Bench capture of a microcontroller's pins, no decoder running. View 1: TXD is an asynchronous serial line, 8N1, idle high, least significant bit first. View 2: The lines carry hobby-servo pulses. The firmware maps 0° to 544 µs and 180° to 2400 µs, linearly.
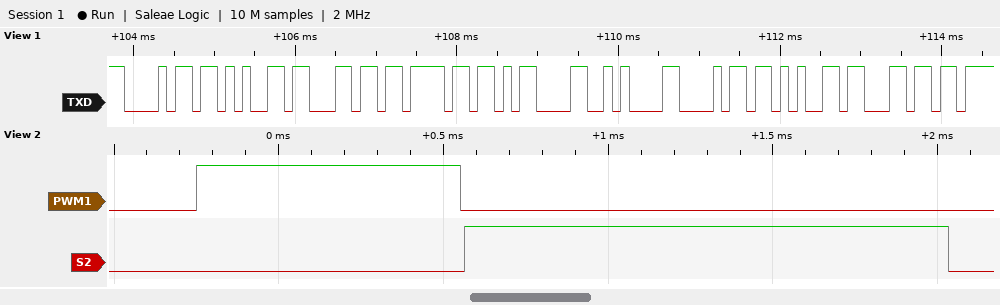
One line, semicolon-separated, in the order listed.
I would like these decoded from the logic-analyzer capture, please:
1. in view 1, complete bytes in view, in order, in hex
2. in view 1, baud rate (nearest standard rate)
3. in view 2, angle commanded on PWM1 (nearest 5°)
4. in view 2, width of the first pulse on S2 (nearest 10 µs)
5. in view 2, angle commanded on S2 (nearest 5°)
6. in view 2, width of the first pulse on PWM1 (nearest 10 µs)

68 65 6C 6F 0D 0A 68 65 6C; 9600 baud; 25°; 1470 µs; 90°; 800 µs
